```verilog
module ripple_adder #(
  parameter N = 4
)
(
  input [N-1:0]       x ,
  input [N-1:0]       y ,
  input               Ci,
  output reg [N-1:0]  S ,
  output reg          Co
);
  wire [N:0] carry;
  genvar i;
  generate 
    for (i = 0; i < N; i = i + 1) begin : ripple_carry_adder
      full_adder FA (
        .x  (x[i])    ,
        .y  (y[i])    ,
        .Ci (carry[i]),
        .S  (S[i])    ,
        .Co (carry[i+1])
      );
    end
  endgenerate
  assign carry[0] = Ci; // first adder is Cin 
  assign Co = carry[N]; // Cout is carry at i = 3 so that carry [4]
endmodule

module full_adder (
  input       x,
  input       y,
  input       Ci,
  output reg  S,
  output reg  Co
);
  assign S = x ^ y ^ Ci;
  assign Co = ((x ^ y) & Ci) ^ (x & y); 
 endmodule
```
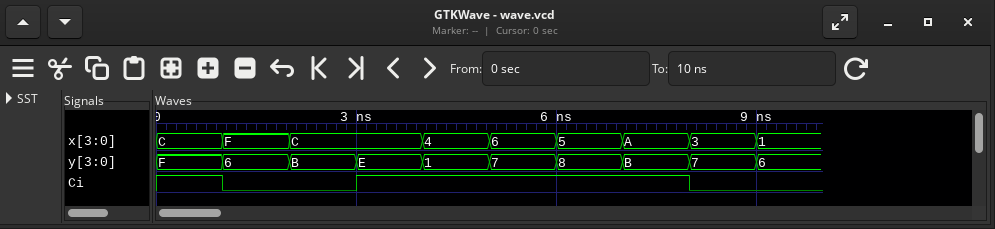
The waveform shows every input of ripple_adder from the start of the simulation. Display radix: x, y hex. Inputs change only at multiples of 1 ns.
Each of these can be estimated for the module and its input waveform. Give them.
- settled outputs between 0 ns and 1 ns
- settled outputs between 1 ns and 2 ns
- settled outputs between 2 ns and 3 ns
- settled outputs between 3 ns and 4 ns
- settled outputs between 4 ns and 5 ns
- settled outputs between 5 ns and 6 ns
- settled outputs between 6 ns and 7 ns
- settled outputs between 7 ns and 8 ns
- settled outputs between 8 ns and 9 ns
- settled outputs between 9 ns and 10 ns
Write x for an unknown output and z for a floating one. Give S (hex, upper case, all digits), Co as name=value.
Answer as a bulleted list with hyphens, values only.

- S=C, Co=1
- S=5, Co=1
- S=7, Co=1
- S=B, Co=1
- S=6, Co=0
- S=E, Co=0
- S=E, Co=0
- S=6, Co=1
- S=A, Co=0
- S=7, Co=0
